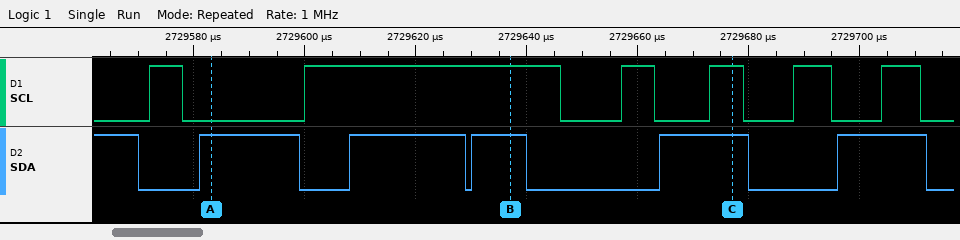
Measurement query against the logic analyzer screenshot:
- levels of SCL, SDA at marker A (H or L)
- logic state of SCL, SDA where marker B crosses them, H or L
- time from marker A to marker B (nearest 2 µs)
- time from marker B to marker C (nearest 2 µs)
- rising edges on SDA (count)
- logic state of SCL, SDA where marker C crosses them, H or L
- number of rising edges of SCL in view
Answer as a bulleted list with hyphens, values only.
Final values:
- SCL=L, SDA=H
- SCL=H, SDA=H
- 54 µs
- 40 µs
- 5
- SCL=H, SDA=H
- 6
